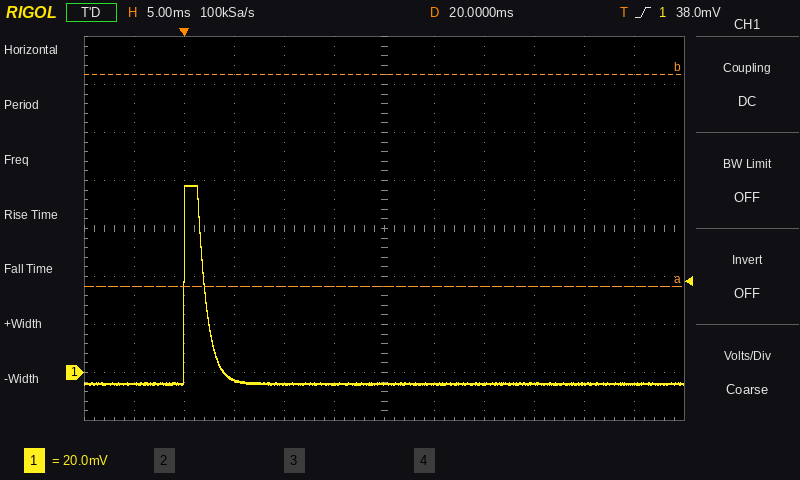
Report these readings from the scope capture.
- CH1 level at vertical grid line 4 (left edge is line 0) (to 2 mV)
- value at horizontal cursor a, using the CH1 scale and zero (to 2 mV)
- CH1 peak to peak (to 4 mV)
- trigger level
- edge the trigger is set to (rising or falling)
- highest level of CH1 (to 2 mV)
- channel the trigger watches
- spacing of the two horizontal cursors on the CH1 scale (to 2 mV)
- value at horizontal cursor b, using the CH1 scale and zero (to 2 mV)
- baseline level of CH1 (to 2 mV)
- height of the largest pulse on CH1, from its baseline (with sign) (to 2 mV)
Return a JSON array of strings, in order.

["-4 mV", "36 mV", "84 mV", "38.0 mV", "rising", "78 mV", "CH1", "88 mV", "124 mV", "-4 mV", "+82 mV"]
